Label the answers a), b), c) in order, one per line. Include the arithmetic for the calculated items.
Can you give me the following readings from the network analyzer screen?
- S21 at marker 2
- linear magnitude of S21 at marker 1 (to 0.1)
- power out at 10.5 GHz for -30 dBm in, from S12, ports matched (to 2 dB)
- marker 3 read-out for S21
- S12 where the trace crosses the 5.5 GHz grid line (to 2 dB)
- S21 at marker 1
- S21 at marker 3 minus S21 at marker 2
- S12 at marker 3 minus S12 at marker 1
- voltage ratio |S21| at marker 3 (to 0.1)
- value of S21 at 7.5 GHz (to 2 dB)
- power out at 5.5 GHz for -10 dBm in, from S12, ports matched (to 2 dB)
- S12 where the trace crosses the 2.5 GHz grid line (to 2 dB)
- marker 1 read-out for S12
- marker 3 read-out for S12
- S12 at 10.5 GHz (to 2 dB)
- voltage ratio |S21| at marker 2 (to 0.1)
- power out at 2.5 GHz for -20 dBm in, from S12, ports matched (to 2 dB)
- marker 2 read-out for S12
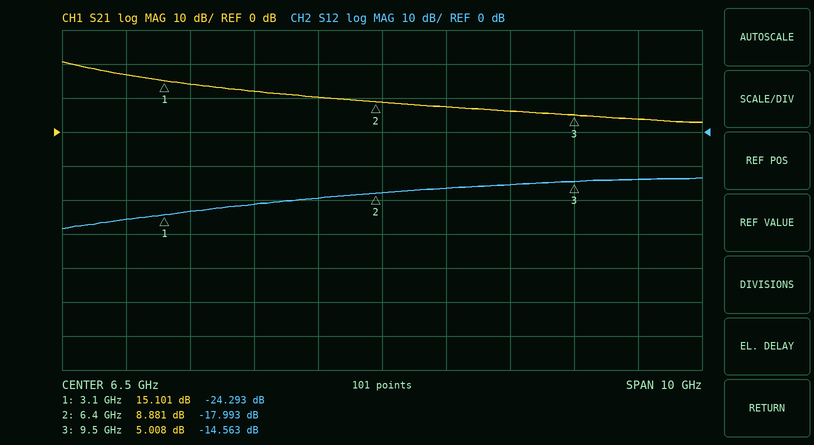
a) 8.881 dB
b) 10^(15.101/20) ≈ 5.7
c) -30 dBm + (-14 dB) = -44 dBm
d) 5.008 dB
e) -20 dB
f) 15.101 dB
g) 5.008 − (8.881) = -3.873 dB
h) -14.563 − (-24.293) = 9.730 dB
i) 10^(5.008/20) ≈ 1.8
j) 8 dB
k) -10 dBm + (-20 dB) = -30 dBm
l) -26 dB
m) -24.293 dB
n) -14.563 dB
o) -14 dB
p) 10^(8.881/20) ≈ 2.8
q) -20 dBm + (-26 dB) = -46 dBm
r) -17.993 dB
